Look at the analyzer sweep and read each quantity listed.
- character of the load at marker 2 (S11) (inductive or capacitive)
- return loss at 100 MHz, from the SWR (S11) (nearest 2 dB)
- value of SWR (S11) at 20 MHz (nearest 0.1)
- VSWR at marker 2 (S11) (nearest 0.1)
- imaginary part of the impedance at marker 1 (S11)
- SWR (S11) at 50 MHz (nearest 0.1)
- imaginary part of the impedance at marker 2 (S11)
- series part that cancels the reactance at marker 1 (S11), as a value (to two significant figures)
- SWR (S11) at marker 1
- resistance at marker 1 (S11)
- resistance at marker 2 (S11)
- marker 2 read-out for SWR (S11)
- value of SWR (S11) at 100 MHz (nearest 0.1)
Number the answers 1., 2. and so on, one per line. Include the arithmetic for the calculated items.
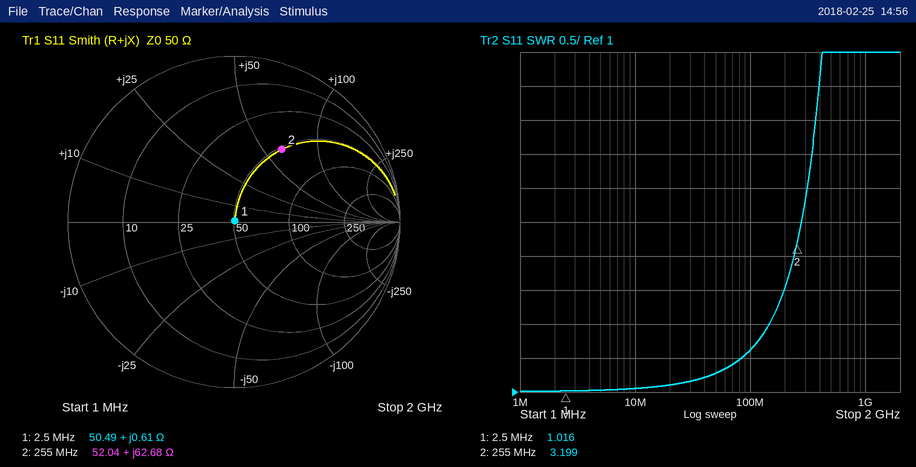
1. inductive
2. −20 log10((1.6 − 1)/(1.6 + 1)) ≈ 12.7 dB, so 12 dB to the nearest 2 dB
3. 1.1
4. 3.2
5. +0.61 Ω
6. 1.3
7. +62.68 Ω
8. C = 1/(2π × 2.5 MHz × 0.61 Ω) ≈ 104 nF, so 100 nF to two significant figures
9. 1.016
10. 50.49 Ω
11. 52.04 Ω
12. 3.199
13. 1.6
